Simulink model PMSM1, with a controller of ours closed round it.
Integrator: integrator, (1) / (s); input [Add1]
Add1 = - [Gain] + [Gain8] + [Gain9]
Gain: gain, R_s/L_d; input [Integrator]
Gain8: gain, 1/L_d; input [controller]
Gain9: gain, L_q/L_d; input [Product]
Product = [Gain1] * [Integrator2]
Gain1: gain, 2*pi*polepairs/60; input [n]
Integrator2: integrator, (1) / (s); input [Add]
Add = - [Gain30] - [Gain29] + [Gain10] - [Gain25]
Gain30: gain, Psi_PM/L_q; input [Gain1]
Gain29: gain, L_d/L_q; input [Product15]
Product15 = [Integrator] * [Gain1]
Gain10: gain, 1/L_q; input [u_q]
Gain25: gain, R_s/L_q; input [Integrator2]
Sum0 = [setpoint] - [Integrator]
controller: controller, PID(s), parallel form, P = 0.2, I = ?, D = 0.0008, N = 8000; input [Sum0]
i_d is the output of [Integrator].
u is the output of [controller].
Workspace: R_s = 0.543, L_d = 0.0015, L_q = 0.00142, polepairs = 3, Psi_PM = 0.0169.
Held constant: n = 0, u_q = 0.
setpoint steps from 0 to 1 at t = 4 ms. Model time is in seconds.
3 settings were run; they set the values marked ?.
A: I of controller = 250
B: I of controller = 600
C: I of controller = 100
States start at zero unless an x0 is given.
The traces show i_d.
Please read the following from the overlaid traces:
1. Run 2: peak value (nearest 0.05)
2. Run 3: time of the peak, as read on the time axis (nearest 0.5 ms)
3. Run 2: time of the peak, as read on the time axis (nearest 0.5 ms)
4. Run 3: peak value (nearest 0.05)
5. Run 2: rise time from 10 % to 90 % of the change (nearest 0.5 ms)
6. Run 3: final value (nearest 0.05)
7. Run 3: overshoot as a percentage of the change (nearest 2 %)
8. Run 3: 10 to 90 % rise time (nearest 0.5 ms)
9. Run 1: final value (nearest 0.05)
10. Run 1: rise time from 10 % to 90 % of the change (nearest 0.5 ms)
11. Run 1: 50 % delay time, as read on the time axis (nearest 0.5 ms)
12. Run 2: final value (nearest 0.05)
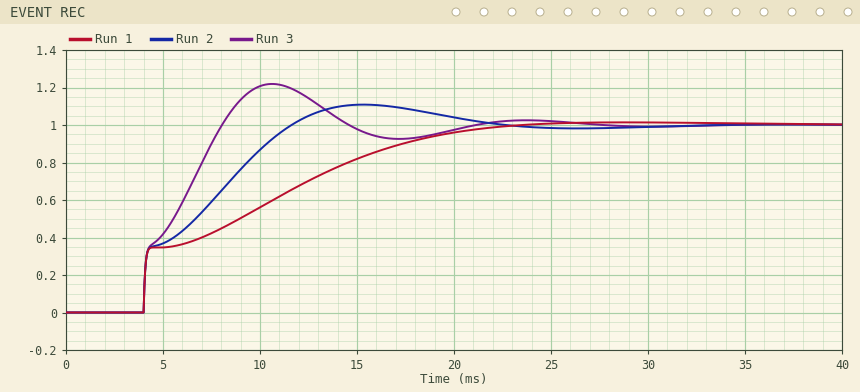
1.10
10.5 ms
15.5 ms
1.20
6.5 ms
1.00
22 %
3.5 ms
1.00
13.5 ms
9.0 ms
1.00
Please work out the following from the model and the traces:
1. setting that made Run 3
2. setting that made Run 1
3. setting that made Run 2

B
C
A
